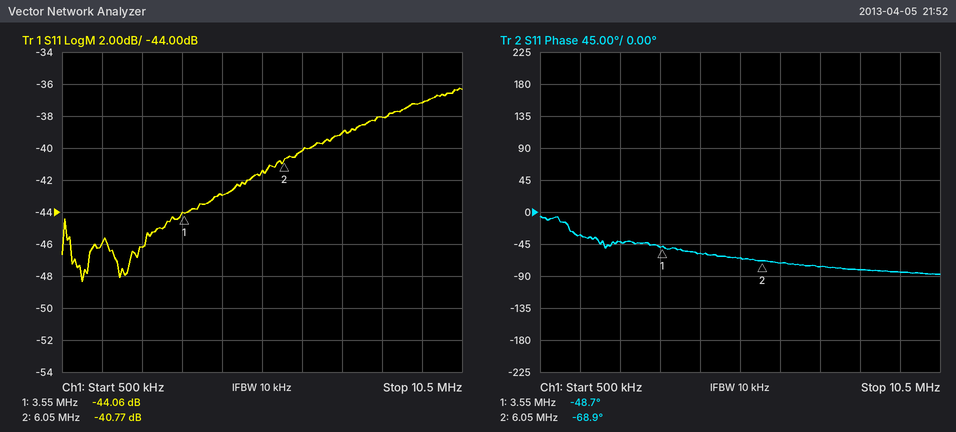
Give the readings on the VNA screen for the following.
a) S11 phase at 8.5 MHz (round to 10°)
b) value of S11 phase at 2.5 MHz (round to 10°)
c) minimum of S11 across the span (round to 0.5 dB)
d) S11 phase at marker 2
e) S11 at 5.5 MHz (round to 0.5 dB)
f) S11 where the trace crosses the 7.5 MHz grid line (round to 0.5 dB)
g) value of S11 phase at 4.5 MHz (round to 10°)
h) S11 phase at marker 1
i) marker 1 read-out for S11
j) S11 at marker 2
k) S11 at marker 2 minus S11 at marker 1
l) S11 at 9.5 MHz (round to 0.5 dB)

-80°
-40°
-48.5 dB
-68.9°
-41.5 dB
-39.0 dB
-60°
-48.7°
-44.06 dB
-40.77 dB
3.29 dB
-37.0 dB
